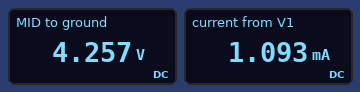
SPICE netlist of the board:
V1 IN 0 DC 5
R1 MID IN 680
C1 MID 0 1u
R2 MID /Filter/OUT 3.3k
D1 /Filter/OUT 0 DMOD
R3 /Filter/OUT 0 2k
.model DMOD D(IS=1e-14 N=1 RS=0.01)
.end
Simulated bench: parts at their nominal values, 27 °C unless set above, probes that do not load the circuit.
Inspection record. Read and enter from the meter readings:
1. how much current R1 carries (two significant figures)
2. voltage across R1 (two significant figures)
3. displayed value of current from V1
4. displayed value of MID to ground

1.1 mA
740 mV
1.093 mA
4.257 V
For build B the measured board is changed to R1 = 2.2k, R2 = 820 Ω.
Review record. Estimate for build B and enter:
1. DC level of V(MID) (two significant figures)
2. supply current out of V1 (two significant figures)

1.8 V
1.4 mA
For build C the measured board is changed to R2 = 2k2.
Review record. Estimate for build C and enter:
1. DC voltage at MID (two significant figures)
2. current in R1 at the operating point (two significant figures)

4.0 V
1.5 mA
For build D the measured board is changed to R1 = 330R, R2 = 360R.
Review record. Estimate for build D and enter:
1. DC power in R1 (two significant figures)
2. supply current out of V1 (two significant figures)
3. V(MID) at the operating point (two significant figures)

13 mW
6.2 mA
2.9 V
